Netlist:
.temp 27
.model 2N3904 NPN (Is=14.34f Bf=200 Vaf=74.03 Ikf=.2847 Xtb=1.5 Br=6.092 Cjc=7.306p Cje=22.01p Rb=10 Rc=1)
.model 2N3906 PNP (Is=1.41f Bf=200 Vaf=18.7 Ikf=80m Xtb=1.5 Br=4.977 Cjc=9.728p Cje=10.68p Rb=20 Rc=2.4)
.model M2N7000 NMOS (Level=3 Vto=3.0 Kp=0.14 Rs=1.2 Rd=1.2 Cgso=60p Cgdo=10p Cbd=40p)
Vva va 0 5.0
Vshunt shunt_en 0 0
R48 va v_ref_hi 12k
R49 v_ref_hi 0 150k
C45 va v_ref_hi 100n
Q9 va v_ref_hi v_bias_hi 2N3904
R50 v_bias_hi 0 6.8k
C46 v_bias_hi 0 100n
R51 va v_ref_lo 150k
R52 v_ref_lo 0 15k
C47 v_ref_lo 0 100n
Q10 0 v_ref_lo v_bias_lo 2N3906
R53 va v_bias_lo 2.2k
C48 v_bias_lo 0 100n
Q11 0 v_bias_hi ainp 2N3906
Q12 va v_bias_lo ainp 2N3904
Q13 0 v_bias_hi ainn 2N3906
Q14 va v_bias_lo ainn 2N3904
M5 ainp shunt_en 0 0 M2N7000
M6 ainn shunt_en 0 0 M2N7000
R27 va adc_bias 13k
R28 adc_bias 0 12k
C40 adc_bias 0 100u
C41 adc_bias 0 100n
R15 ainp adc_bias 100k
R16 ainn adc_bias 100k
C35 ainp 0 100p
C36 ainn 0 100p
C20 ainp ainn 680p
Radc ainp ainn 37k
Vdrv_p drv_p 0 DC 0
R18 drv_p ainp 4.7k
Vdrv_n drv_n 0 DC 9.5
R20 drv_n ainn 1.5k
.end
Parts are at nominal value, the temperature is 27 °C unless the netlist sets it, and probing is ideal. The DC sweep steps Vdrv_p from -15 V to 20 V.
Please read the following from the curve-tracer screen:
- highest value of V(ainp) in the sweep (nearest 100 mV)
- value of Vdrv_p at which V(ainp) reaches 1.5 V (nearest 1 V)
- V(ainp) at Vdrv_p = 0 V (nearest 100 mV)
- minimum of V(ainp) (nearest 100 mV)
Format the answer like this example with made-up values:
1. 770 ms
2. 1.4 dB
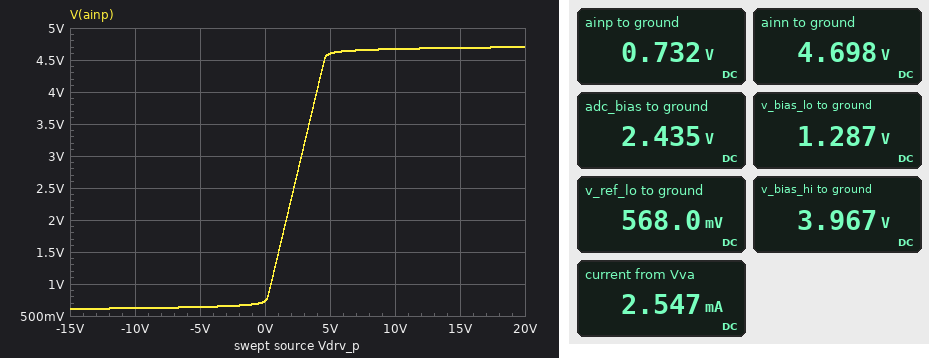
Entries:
1. 4.7 V
2. 1 V
3. 700 mV
4. 600 mV
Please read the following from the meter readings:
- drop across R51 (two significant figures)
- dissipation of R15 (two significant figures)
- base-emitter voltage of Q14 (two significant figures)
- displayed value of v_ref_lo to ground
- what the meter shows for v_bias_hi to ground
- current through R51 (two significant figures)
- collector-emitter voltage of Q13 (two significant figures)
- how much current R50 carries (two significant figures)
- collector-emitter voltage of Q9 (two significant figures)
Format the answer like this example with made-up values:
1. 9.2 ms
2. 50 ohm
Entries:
1. 4.4 V
2. 29 µW
3. -3.4 V
4. 568.0 mV
5. 3.967 V
6. 30 µA
7. -4.7 V
8. 580 µA
9. 1.0 V
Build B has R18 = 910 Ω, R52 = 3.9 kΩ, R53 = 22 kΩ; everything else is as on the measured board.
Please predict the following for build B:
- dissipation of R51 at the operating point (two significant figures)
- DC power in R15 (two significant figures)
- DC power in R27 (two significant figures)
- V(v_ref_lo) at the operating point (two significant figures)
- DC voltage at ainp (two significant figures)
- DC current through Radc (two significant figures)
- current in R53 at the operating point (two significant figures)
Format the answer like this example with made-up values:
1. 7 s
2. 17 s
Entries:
1. 160 µW
2. 48 µW
3. 520 µW
4. 130 mV
5. 210 mV
6. 120 µA
7. 190 µA
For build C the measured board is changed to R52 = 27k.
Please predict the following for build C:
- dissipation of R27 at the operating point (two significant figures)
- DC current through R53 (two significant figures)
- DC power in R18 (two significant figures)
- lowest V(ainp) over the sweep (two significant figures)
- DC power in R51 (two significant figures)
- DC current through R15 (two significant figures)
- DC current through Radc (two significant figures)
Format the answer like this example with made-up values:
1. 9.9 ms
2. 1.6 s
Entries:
1. 500 µW
2. 1.5 mA
3. 240 µW
4. 970 mV
5. 110 µW
6. 14 µA
7. 98 µA
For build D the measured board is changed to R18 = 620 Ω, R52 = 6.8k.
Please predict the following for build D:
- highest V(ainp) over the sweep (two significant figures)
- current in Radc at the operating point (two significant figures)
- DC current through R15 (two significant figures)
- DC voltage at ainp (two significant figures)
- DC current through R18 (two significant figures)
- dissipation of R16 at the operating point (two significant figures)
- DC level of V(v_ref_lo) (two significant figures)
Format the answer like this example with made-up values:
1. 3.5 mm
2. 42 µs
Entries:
1. 4.8 V
2. 120 µA
3. 20 µA
4. 370 mV
5. 600 µA
6. 52 µW
7. 280 mV
